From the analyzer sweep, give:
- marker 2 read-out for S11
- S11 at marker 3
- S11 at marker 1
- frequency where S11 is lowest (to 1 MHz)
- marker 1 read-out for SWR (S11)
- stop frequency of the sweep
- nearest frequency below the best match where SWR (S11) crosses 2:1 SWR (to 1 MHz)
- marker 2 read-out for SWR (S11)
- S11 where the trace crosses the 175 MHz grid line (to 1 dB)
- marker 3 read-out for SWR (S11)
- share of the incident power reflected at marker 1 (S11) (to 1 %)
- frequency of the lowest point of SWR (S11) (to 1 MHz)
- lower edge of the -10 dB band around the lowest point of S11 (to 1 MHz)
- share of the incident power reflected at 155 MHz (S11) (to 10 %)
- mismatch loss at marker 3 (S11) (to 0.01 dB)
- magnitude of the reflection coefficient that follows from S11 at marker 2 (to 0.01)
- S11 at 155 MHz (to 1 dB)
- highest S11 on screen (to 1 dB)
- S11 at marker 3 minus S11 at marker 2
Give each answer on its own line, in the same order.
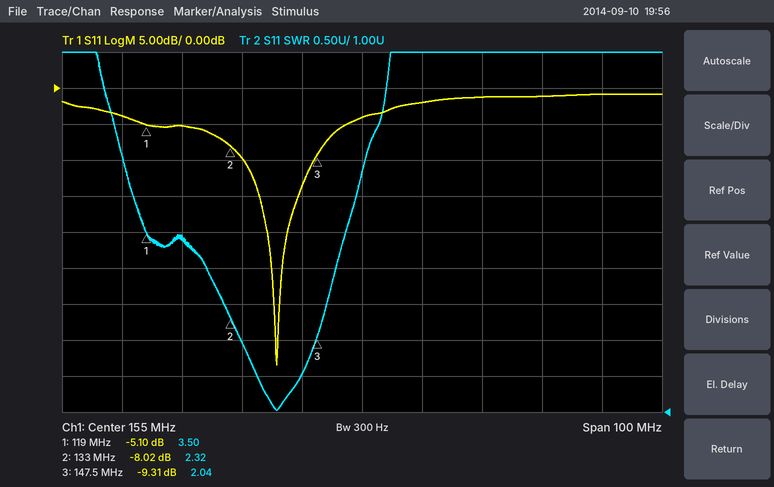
-8.02 dB
-9.31 dB
-5.10 dB
141 MHz
3.50
205 MHz
135 MHz
2.32
-1 dB
2.04
31 %
141 MHz
135 MHz
40 %
0.54 dB
0.40
-4 dB
-1 dB
-1.29 dB
